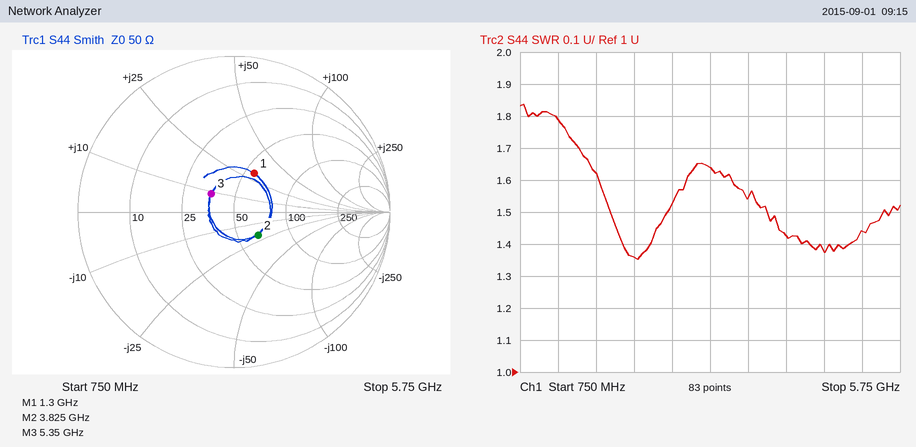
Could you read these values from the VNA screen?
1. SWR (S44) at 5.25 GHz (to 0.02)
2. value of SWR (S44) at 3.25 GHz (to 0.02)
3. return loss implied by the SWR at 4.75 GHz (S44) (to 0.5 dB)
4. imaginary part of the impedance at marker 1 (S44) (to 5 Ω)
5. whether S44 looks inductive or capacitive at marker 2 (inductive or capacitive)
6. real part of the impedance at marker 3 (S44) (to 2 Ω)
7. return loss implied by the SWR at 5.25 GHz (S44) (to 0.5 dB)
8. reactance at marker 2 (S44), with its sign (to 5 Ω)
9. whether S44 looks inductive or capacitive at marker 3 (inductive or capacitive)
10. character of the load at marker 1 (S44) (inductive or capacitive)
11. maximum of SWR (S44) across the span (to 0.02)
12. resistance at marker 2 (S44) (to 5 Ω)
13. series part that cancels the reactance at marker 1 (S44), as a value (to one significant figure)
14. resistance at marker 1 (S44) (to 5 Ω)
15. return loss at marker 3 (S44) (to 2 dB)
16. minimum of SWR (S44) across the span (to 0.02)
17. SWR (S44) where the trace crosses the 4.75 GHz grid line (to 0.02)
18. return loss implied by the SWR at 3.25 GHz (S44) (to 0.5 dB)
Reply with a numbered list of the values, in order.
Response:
1. 1.44
2. 1.64
3. 16.0 dB
4. +30 Ω
5. capacitive
6. 36 Ω
7. 15.0 dB
8. -20 Ω
9. inductive
10. inductive
11. 1.84
12. 65 Ω
13. 4 pF
14. 55 Ω
15. 14 dB
16. 1.36
17. 1.38
18. 12.5 dB
